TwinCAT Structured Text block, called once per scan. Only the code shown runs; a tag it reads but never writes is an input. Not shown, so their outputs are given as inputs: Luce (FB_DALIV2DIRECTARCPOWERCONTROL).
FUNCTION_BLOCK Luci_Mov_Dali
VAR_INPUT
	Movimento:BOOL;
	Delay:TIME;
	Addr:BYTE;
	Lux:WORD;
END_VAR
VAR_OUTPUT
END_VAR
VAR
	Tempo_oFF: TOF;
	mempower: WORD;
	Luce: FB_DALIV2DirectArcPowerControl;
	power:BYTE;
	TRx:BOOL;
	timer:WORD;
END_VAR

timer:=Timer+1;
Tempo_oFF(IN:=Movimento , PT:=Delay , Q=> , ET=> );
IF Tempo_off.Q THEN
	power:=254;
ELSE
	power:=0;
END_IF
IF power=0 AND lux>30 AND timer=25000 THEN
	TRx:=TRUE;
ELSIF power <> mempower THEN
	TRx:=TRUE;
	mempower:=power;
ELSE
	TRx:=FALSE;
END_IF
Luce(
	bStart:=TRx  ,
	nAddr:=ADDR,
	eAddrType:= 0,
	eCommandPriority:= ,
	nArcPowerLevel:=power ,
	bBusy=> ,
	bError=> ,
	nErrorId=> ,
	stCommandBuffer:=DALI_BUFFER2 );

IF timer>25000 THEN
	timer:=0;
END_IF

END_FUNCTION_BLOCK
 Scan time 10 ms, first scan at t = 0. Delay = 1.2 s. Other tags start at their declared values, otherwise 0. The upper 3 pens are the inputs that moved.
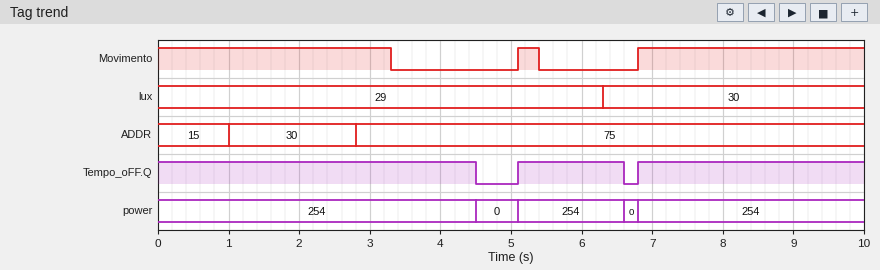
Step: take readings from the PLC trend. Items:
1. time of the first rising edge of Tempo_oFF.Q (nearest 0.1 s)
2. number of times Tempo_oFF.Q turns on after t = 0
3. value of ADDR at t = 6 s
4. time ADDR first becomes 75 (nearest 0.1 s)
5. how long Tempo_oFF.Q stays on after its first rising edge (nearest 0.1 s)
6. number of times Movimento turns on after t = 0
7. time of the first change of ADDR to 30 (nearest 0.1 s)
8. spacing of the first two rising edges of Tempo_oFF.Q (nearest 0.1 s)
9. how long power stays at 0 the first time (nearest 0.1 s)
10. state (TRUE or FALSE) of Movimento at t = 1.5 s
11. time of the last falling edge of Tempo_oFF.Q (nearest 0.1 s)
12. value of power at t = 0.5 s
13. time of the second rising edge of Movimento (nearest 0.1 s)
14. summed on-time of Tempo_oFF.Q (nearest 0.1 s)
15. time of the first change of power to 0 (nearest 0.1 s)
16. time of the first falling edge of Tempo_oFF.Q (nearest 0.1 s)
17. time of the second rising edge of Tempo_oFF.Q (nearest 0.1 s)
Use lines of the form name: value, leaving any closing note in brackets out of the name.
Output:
time of the first rising edge of Tempo_oFF.Q: 5.1 s
number of times Tempo_oFF.Q turns on after t = 0: 2
value of ADDR at t = 6 s: 75
time ADDR first becomes 75: 2.8 s
how long Tempo_oFF.Q stays on after its first rising edge: 1.5 s
number of times Movimento turns on after t = 0: 2
time of the first change of ADDR to 30: 1.0 s
spacing of the first two rising edges of Tempo_oFF.Q: 1.7 s
how long power stays at 0 the first time: 0.6 s
state (TRUE or FALSE) of Movimento at t = 1.5 s: TRUE
time of the last falling edge of Tempo_oFF.Q: 6.6 s
value of power at t = 0.5 s: 254
time of the second rising edge of Movimento: 6.8 s
summed on-time of Tempo_oFF.Q: 9.2 s
time of the first change of power to 0: 4.5 s
time of the first falling edge of Tempo_oFF.Q: 4.5 s
time of the second rising edge of Tempo_oFF.Q: 6.8 s
